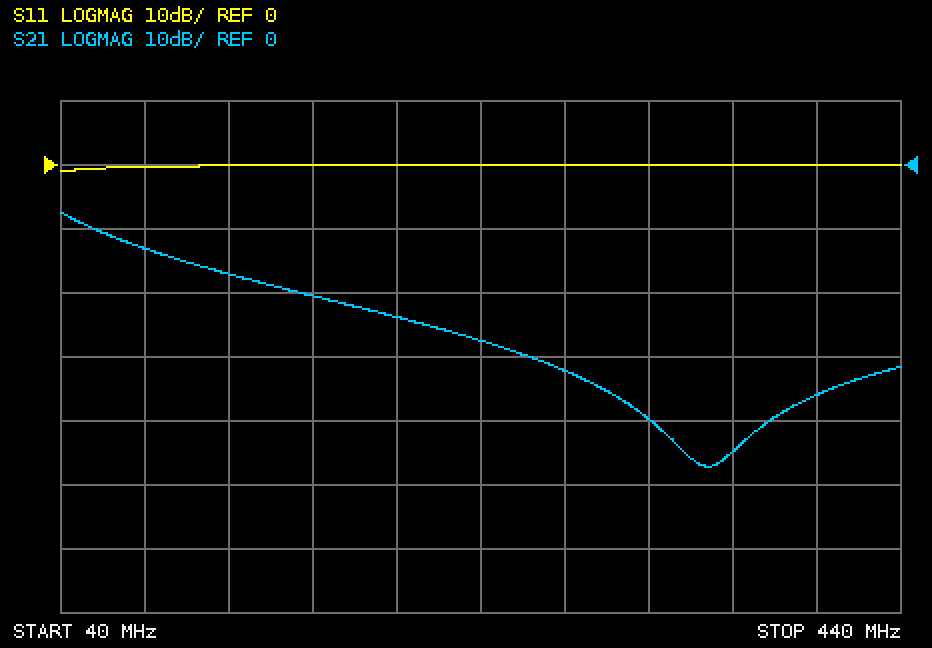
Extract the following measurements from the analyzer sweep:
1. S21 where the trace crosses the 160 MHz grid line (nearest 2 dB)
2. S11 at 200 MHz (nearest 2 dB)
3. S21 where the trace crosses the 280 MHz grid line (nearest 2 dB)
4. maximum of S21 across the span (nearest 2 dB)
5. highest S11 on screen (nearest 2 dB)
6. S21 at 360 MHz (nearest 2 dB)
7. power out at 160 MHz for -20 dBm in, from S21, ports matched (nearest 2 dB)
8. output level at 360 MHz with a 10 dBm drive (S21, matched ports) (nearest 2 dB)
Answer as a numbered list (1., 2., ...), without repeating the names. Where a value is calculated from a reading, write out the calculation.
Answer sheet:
1. -20 dB
2. 0 dB
3. -32 dB
4. -8 dB
5. 0 dB
6. -44 dB
7. -20 dBm + (-20 dB) = -40 dBm
8. 10 dBm + (-44 dB) = -34 dBm
